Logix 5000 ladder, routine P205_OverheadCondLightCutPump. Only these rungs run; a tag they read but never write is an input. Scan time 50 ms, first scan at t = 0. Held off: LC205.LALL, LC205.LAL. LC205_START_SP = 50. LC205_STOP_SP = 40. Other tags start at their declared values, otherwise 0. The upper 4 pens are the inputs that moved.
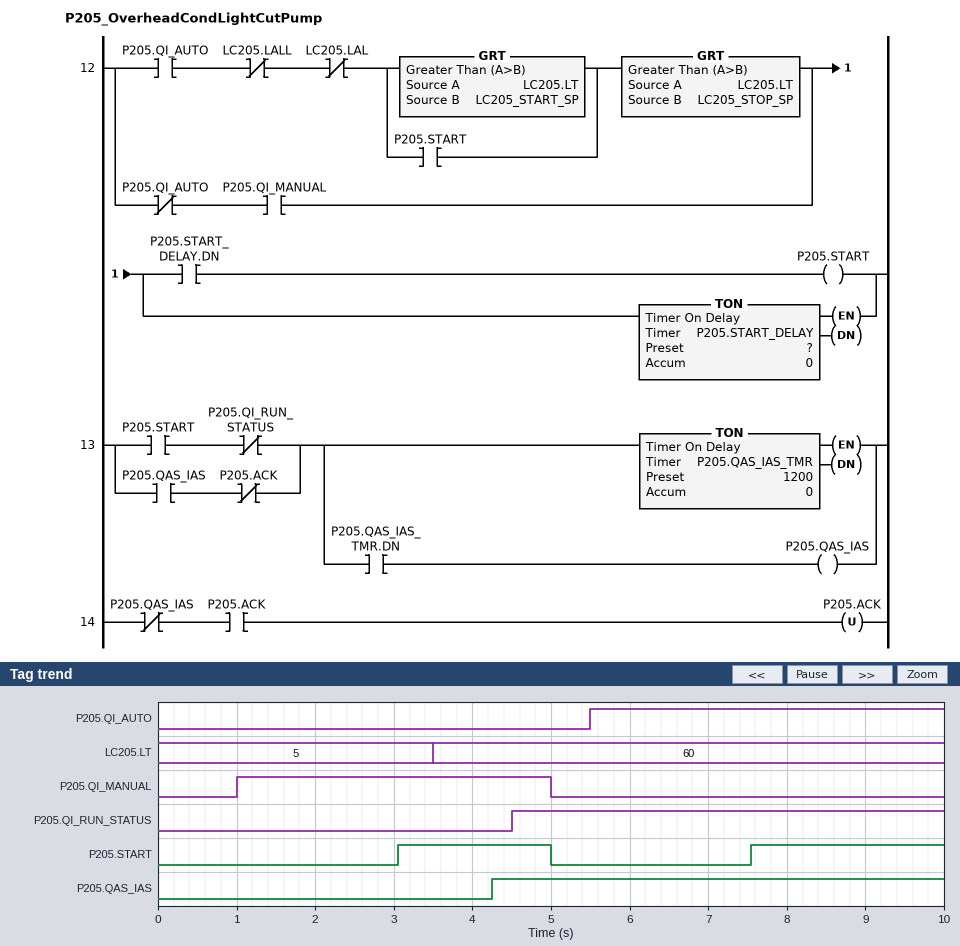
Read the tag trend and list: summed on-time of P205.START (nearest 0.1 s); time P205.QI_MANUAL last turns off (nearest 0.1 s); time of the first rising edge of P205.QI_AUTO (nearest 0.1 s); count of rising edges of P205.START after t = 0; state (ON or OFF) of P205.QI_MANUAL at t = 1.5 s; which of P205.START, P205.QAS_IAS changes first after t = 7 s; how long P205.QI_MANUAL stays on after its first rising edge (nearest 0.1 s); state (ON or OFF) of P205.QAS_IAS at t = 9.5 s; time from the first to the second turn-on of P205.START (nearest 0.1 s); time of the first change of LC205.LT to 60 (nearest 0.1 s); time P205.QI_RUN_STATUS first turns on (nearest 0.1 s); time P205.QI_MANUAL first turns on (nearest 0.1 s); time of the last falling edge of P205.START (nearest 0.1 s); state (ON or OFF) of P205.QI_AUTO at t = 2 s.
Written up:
4.4 s
5.0 s
5.5 s
2
ON
P205.START
4.0 s
ON
4.5 s
3.5 s
4.5 s
1.0 s
5.0 s
OFF
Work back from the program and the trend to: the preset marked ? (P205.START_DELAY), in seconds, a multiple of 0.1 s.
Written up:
2.0 s
